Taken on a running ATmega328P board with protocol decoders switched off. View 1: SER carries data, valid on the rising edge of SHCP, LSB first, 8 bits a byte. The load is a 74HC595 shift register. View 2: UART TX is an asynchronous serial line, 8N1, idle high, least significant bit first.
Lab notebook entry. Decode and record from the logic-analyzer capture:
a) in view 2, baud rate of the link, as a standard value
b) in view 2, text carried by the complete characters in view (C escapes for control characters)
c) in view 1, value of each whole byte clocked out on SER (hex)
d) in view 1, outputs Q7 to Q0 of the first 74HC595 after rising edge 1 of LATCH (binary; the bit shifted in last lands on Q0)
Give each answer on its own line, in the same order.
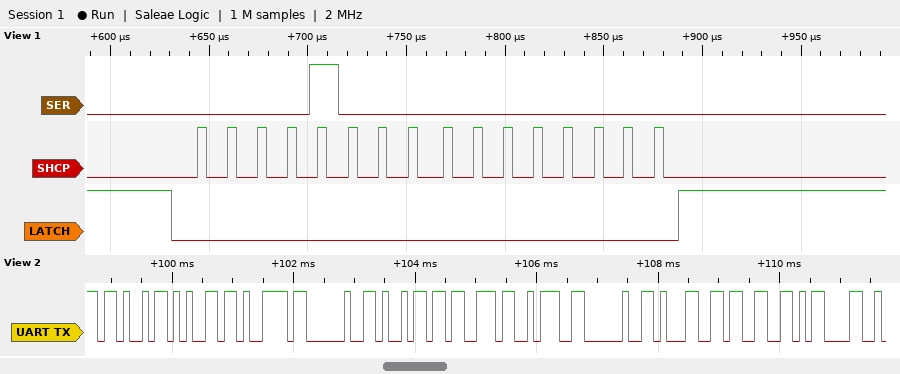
9600 baud
"Key is: 13\r"
10 00
00000000
